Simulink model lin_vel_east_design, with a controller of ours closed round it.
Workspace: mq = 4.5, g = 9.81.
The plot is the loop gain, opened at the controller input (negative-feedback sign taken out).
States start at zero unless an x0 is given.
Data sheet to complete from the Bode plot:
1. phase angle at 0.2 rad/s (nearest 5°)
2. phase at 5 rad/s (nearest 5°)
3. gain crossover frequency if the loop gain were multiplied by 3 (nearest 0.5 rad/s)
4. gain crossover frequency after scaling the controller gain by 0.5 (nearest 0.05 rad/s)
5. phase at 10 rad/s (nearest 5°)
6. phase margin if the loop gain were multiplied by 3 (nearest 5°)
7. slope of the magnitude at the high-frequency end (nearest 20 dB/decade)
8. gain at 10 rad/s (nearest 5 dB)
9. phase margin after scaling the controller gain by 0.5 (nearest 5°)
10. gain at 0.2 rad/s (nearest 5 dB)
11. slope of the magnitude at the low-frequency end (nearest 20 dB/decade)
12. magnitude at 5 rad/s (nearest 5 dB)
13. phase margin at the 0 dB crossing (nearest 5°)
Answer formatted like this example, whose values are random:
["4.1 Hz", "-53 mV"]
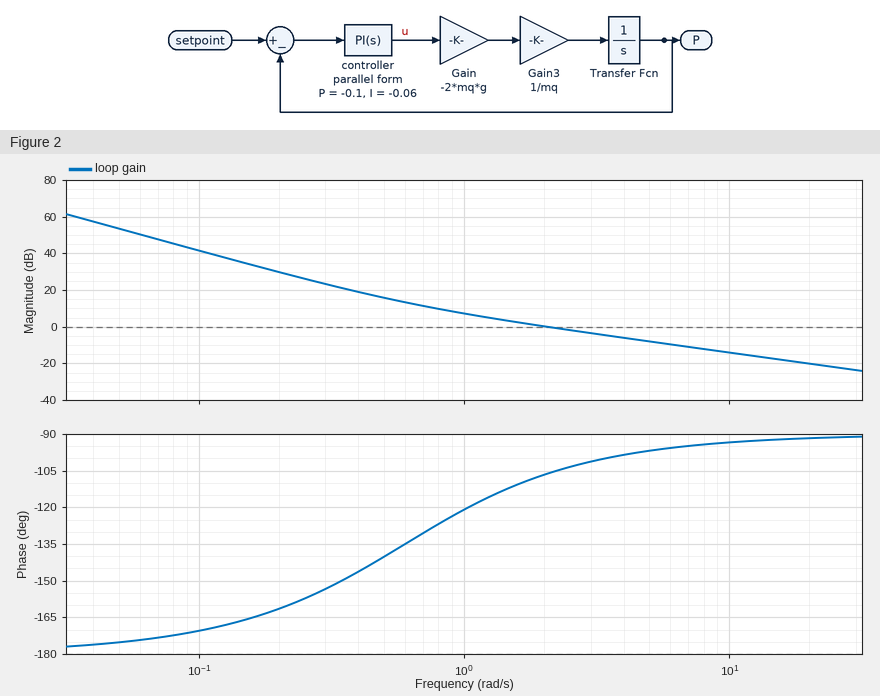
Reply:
["-160°", "-95°", "6.0 rad/s", "1.10 rad/s", "-95°", "85°", "-20 dB/decade", "-15 dB", "60°", "30 dB", "-40 dB/decade", "-10 dB", "75°"]
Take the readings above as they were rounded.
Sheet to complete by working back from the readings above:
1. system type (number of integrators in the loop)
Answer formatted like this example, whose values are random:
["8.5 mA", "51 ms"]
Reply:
["2"]
